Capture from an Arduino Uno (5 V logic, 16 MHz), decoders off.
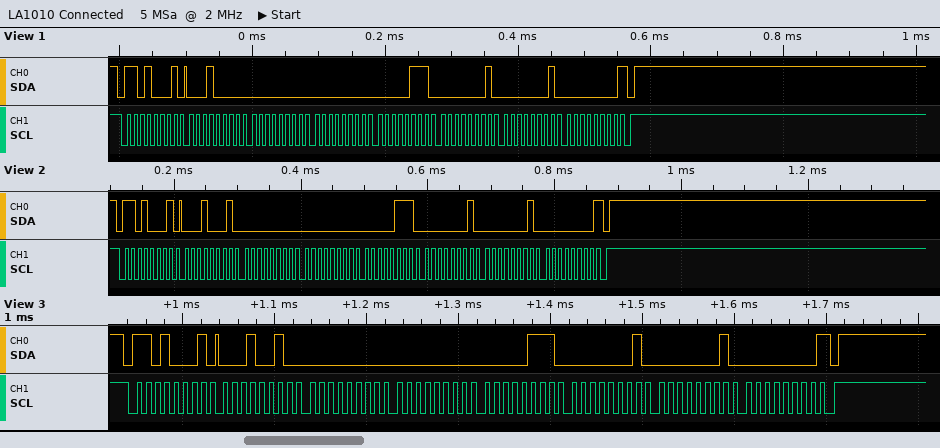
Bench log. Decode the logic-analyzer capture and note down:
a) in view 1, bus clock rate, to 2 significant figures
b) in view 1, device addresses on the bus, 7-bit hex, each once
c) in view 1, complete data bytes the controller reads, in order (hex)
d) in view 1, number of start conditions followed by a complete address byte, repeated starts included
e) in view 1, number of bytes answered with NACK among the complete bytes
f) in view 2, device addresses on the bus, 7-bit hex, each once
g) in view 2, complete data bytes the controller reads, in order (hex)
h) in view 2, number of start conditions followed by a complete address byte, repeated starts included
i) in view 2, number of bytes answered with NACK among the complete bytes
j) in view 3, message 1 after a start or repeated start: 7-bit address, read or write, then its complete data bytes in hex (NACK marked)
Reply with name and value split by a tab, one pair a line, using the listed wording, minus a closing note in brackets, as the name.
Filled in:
in view 1, bus clock rate, to 2 significant figures	100 kHz
in view 1, device addresses on the bus, 7-bit hex, each once	0x68
in view 1, complete data bytes the controller reads, in order	10 00 00 07 01 01 00
in view 1, number of start conditions followed by a complete address byte, repeated starts included	1
in view 1, number of bytes answered with NACK among the complete bytes	1
in view 2, device addresses on the bus, 7-bit hex, each once	0x68
in view 2, complete data bytes the controller reads, in order	11 00 00 07 01 01 00
in view 2, number of start conditions followed by a complete address byte, repeated starts included	1
in view 2, number of bytes answered with NACK among the complete bytes	1
in view 3, message 1 after a start or repeated start: 7-bit address, read or write, then its complete data bytes in hex	0x68 read: 12 00 00 07 01 01 00 NACK
